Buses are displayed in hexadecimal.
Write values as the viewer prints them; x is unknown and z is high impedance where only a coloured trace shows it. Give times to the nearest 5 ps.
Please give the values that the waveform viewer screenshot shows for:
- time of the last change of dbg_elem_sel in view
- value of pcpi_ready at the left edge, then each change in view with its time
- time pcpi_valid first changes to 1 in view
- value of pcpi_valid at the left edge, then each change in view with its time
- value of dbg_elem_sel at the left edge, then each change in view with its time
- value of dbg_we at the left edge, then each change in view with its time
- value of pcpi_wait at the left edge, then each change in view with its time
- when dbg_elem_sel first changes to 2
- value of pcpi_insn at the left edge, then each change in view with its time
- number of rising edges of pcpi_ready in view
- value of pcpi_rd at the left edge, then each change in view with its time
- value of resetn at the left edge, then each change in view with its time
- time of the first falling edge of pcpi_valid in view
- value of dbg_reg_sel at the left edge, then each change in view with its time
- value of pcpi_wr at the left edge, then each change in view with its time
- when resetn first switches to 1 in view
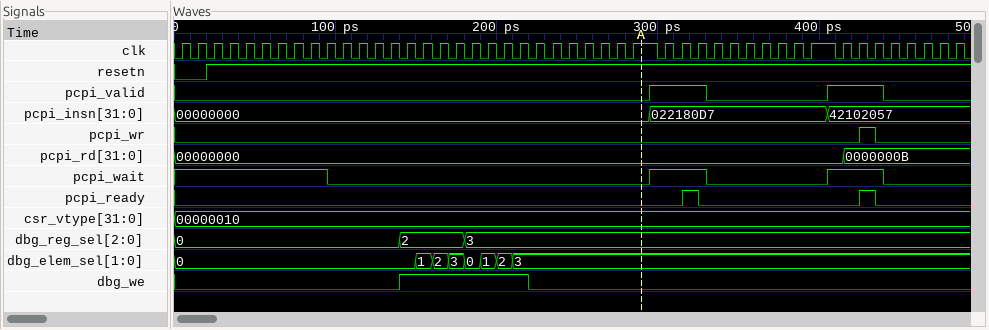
210 ps
0, 1 at 315 ps, 0 at 325 ps, 1 at 425 ps, 0 at 435 ps
295 ps
0, 1 at 295 ps, 0 at 330 ps, 1 at 405 ps, 0 at 440 ps
0, 1 at 150 ps, 2 at 160 ps, 3 at 170 ps, 0 at 180 ps, 1 at 190 ps, 2 at 200 ps, 3 at 210 ps
0, 1 at 140 ps, 0 at 220 ps
1, 0 at 95 ps, 1 at 295 ps, 0 at 330 ps, 1 at 405 ps, 0 at 440 ps
160 ps
00000000, 022180D7 at 295 ps, 42102057 at 405 ps
2
00000000, 0000000B at 415 ps
0, 1 at 20 ps
330 ps
0, 2 at 140 ps, 3 at 180 ps
0, 1 at 425 ps, 0 at 435 ps
20 ps
